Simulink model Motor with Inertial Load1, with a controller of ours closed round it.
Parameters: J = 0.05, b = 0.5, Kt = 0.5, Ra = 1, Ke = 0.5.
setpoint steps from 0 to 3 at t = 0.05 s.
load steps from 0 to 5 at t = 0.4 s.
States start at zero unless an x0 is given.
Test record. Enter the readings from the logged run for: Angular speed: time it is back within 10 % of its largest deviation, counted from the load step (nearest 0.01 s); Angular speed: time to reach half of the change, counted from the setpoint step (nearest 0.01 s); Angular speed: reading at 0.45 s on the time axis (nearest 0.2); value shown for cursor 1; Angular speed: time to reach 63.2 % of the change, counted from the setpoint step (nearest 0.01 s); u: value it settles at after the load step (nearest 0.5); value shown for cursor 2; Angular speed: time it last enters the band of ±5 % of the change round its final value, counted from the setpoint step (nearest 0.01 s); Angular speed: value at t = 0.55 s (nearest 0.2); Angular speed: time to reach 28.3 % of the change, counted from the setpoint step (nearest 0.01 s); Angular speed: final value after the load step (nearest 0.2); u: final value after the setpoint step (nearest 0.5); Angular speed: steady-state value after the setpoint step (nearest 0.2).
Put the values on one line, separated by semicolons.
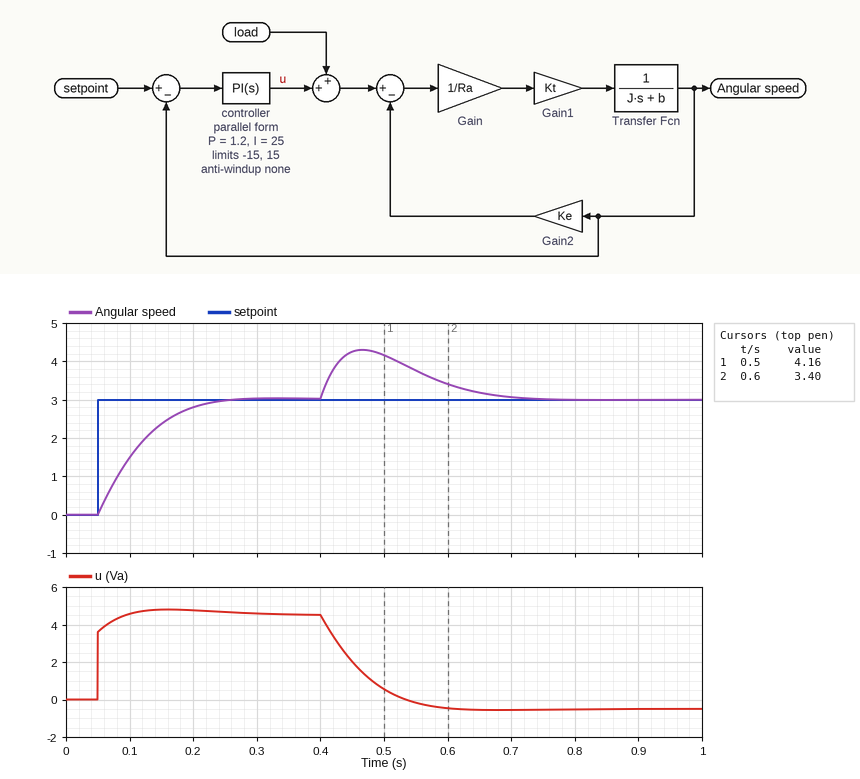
0.27 s; 0.05 s; 4.2; 4.16; 0.07 s; -0.5; 3.40; 0.16 s; 3.8; 0.03 s; 3.0; 4.5; 3.0
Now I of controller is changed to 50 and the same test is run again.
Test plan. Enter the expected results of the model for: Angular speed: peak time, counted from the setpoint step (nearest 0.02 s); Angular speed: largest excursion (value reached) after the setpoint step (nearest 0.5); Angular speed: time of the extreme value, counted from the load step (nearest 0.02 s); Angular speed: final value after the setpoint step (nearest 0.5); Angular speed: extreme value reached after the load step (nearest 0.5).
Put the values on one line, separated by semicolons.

0.14 s; 3.5; 0.06 s; 3.0; 4.0
